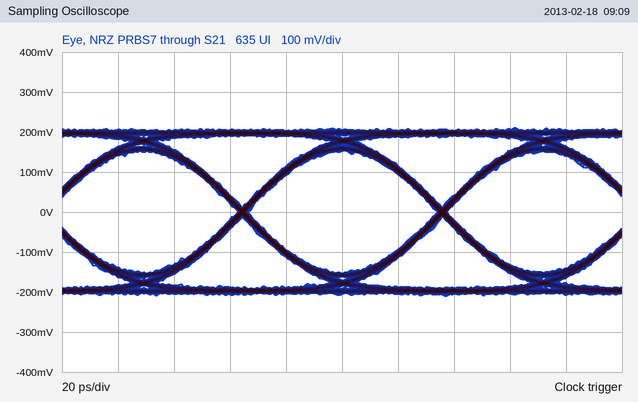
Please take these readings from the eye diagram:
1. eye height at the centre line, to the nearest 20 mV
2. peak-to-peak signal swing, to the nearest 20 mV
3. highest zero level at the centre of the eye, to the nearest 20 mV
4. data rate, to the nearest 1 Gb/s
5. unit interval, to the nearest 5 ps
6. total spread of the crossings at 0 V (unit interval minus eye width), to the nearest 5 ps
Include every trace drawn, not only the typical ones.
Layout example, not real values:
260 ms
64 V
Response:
300 mV
420 mV
-160 mV
14 Gb/s
70 ps
5 ps
